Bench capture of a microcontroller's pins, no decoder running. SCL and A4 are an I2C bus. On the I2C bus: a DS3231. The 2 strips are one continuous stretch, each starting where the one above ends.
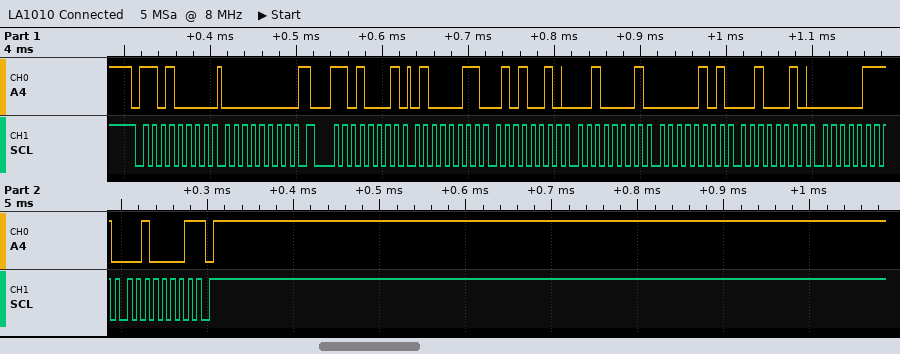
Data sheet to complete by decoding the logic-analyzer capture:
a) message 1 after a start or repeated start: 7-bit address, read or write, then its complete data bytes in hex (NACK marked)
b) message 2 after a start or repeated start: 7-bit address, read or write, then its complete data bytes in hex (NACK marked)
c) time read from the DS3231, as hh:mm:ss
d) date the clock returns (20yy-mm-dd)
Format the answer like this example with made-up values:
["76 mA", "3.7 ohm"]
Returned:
["0x68 write: 00", "0x68 read: 43 52 21 05 22 07 21 NACK", "21:52:43", "2021-07-22"]
